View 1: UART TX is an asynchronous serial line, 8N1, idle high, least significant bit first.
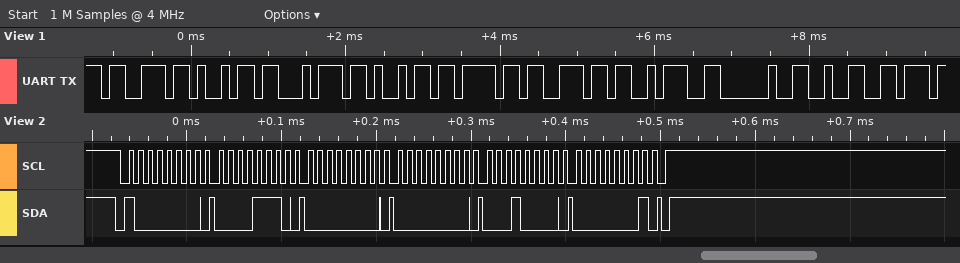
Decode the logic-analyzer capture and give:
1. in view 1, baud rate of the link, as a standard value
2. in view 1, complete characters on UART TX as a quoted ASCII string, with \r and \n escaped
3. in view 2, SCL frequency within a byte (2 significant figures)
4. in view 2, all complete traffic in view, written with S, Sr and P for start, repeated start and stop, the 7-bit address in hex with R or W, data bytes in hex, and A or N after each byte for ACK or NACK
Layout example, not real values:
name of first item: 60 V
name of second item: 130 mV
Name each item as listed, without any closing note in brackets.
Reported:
in view 1, baud rate of the link, as a standard value: 9600 baud
in view 1, complete characters on UART TX as a quoted ASCII string, with \r and \n escaped: "sition: 2"
in view 2, SCL frequency within a byte: 100 kHz
in view 2, all complete traffic in view, written with S, Sr and P for start, repeated start and stop, the 7-bit address in hex with R or W, data bytes in hex, and A or N after each byte for ACK or NACK: S 40W A 0E A 00 A 00 A 10 A 01 A P
